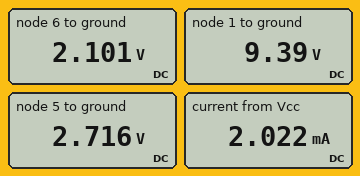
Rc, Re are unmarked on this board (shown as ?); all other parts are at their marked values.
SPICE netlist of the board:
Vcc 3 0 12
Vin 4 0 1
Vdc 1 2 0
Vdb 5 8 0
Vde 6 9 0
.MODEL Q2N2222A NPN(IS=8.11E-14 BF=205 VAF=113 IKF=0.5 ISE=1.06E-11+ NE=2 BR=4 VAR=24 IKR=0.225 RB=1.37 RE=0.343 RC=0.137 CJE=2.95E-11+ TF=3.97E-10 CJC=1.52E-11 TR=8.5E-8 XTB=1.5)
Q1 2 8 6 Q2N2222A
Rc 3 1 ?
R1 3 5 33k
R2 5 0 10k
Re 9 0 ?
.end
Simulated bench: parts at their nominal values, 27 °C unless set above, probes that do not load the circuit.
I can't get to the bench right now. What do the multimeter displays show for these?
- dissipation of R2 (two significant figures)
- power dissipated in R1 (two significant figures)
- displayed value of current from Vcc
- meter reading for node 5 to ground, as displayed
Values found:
740 µW
2.6 mW
2.022 mA
2.716 V
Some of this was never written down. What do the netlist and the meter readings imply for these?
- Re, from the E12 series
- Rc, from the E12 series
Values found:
1.2 kΩ
1.5 kΩ
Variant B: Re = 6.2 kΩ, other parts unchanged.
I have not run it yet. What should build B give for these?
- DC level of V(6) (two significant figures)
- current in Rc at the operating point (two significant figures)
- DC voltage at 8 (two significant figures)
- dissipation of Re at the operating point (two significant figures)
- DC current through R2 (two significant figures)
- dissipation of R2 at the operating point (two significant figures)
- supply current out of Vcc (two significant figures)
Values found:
2.2 V
350 µA
2.8 V
780 µW
280 µA
770 µW
630 µA
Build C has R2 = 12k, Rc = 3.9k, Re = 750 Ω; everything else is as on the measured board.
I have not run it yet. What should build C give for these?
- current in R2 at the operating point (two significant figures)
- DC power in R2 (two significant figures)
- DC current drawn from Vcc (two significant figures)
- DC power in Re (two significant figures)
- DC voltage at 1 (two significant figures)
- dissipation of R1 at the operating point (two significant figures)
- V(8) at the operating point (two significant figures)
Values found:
220 µA
560 µW
2.8 mA
5.2 mW
2.0 V
2.7 mW
2.6 V
